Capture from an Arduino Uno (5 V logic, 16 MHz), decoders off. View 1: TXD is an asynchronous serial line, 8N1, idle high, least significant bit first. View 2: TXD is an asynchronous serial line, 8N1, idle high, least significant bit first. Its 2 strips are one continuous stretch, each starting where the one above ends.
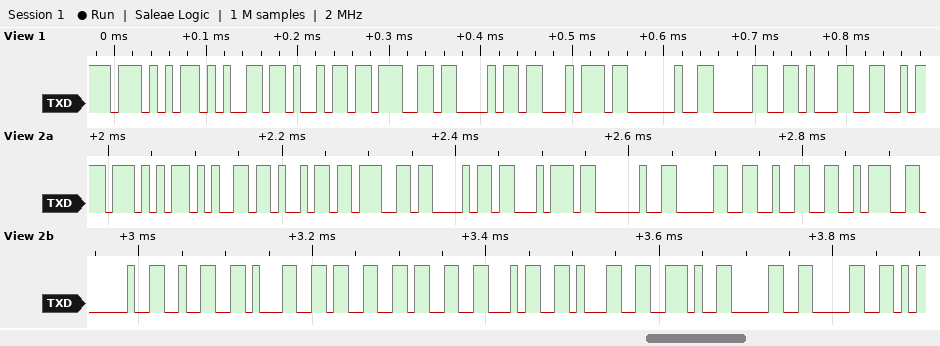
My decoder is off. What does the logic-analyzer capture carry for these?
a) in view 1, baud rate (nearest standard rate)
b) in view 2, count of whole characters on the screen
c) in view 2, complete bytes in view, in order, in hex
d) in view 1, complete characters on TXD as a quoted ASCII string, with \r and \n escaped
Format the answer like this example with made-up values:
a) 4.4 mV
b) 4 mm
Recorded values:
a) 115200 baud
b) 20
c) 57 65 69 67 68 74 20 30 32 3A 20 32 31 33 33 34 31 2E 30 30
d) "Weight 01"
